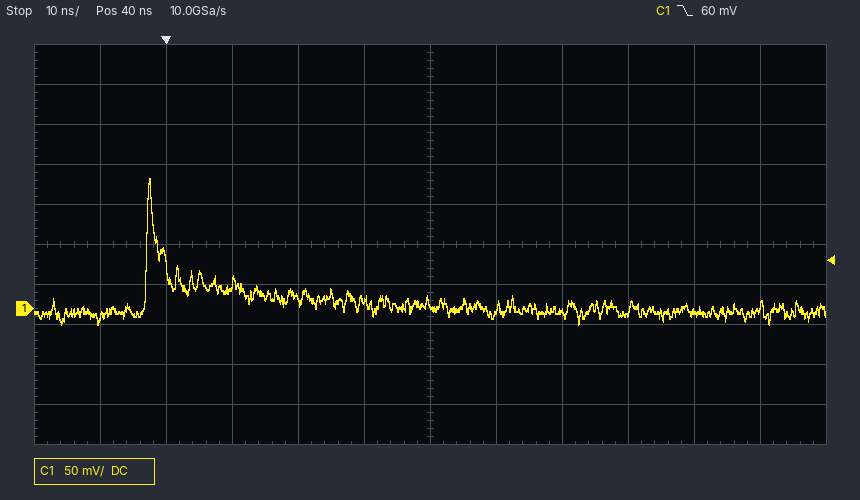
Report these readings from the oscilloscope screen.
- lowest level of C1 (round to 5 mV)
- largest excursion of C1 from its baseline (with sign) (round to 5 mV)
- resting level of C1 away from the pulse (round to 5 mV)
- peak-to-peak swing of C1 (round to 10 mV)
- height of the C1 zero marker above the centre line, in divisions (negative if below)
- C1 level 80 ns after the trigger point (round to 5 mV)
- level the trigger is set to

-20 mV
+165 mV
0 mV
180 mV
-1.6 div
-5 mV
60 mV
